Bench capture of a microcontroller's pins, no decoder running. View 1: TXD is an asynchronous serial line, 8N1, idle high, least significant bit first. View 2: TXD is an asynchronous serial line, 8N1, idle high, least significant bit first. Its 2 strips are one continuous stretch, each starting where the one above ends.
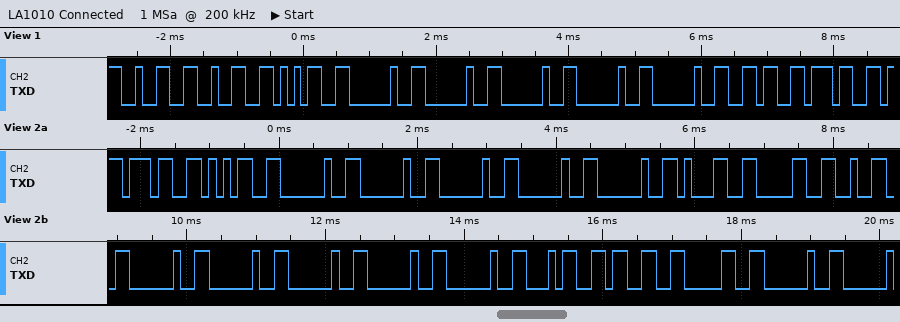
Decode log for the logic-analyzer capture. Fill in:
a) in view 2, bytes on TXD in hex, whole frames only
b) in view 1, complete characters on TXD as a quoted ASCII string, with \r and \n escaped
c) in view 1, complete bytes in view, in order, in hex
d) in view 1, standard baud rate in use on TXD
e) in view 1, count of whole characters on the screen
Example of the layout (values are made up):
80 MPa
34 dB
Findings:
0x37 0x35 0x20 0x20 0x20 0x20 0x20 0x31 0x30 0x32 0x20 0x20 0x20 0x20 0x20 0x34 0x33 0x30 0x20
"225     67"
32 32 35 20 20 20 20 20 36 37
9600 baud
10
